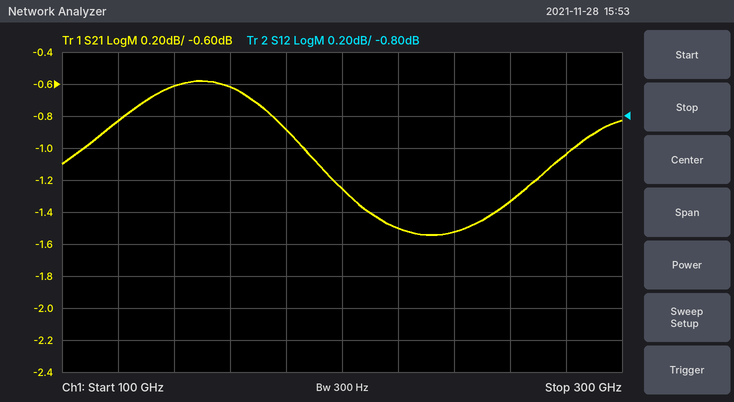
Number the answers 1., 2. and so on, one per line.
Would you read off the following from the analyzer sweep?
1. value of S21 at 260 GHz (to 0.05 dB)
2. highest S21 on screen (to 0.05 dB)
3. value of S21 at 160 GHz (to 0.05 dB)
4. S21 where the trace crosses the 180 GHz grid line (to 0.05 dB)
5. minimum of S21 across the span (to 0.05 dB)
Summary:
1. -1.35 dB
2. -0.60 dB
3. -0.60 dB
4. -0.90 dB
5. -1.55 dB
